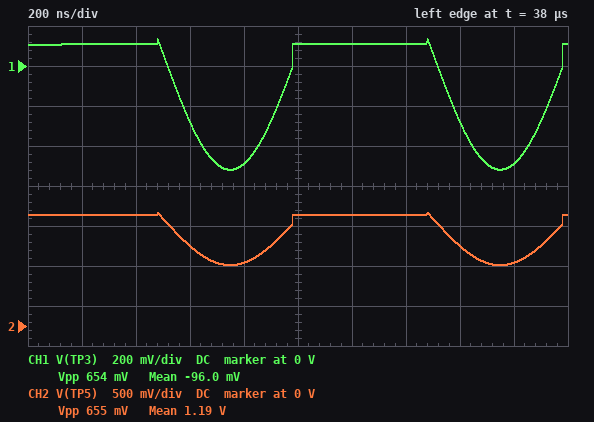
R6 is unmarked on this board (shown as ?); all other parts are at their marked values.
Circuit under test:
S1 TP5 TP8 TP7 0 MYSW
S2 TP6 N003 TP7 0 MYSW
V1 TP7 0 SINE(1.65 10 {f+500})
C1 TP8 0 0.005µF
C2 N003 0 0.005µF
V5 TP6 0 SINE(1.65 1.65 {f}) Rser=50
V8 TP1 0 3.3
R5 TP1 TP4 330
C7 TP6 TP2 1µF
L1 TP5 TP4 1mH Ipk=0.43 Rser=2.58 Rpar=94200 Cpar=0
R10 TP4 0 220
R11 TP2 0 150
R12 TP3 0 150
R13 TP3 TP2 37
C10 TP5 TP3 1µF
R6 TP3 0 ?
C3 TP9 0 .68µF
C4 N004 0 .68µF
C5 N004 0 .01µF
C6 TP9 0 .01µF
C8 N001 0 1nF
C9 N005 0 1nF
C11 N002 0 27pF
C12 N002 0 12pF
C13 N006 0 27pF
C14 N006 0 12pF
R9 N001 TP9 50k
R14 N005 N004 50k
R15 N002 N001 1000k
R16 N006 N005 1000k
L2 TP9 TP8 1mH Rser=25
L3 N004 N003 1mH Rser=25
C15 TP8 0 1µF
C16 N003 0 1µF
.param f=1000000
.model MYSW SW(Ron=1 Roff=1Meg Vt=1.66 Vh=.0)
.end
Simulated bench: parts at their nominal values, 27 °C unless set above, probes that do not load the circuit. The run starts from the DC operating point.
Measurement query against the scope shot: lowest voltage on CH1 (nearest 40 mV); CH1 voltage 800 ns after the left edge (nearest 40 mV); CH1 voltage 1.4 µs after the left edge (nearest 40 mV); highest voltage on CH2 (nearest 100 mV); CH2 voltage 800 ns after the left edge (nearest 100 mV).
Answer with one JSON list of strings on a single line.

["-520 mV", "-480 mV", "120 mV", "1.4 V", "800 mV"]
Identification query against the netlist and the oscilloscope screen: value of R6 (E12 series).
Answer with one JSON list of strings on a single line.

["120 Ω"]
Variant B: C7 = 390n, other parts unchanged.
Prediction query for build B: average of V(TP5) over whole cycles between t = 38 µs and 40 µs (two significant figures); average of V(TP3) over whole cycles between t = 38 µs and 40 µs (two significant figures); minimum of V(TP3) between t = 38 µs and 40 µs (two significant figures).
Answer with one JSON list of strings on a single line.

["1.2 V", "-78 mV", "-500 mV"]
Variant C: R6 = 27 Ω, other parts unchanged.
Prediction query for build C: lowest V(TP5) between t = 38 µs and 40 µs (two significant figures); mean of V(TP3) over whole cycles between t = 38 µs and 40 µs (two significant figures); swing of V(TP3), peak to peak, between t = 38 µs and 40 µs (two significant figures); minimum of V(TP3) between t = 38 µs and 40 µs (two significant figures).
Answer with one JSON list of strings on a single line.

["1.0 V", "-36 mV", "350 mV", "-260 mV"]
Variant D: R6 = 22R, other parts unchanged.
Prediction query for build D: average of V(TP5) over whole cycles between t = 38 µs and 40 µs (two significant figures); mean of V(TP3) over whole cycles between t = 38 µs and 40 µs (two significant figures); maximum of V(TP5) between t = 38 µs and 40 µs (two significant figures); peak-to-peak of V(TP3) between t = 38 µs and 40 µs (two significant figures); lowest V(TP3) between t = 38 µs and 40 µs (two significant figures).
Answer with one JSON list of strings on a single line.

["1.3 V", "-29 mV", "1.4 V", "310 mV", "-230 mV"]
